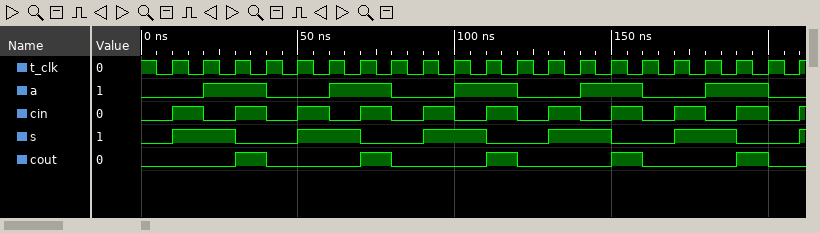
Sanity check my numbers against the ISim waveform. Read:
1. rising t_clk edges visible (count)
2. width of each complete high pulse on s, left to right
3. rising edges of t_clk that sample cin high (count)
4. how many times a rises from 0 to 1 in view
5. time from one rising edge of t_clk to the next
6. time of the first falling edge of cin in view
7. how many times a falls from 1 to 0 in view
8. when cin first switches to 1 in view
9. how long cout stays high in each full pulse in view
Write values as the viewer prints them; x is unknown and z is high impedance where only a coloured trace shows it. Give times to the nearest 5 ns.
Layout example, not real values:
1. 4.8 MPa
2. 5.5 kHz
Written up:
1. 21
2. 20 ns, 20 ns, 20 ns, 20 ns, 20 ns
3. 10
4. 5
5. 10 ns
6. 20 ns
7. 5
8. 10 ns
9. 10 ns, 10 ns, 10 ns, 10 ns, 10 ns
